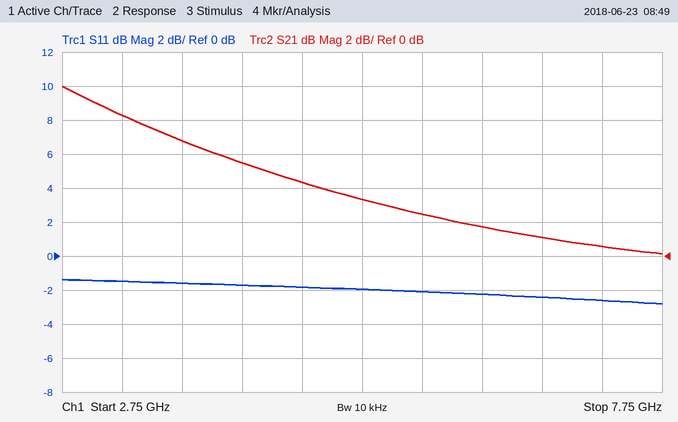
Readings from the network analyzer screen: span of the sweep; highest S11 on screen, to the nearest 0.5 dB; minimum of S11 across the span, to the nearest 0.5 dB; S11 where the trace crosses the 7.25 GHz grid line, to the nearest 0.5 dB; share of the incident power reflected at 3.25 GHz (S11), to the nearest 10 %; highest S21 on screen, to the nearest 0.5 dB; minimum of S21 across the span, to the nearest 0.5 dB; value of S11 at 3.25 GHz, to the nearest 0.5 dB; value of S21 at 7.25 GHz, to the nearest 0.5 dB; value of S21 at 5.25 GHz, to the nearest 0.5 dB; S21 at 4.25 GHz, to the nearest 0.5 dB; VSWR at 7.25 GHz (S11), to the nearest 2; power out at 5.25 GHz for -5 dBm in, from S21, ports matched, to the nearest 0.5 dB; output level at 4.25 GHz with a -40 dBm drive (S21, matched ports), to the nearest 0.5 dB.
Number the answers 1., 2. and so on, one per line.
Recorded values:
1. 5 GHz
2. -1.5 dB
3. -3.0 dB
4. -2.5 dB
5. 70 %
6. 10.0 dB
7. 0.0 dB
8. -1.5 dB
9. 0.5 dB
10. 3.5 dB
11. 5.5 dB
12. 6
13. -1.5 dBm
14. -34.5 dBm
